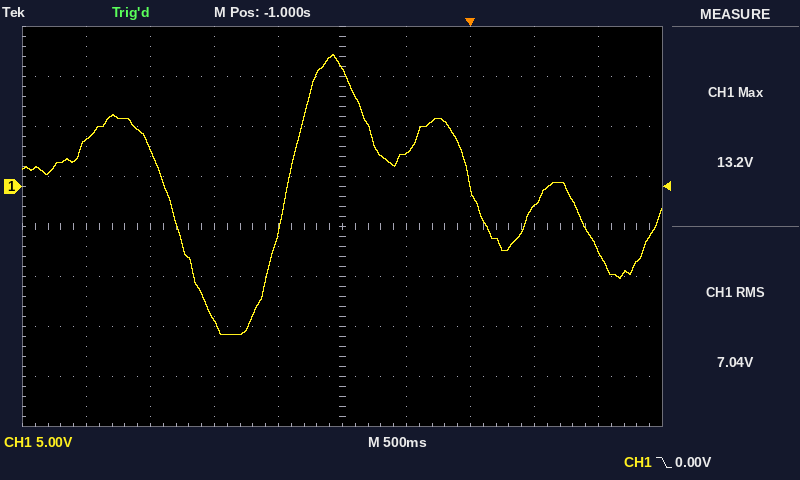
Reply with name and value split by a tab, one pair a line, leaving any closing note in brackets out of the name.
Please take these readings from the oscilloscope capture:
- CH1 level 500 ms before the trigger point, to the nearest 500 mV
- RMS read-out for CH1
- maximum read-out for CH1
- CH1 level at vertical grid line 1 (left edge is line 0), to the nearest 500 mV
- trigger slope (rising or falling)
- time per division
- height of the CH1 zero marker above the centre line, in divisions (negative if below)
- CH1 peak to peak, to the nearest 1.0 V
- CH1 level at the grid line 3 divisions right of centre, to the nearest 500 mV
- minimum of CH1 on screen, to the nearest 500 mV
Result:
CH1 level 500 ms before the trigger point, to the nearest 500 mV	3.5 V
RMS read-out for CH1	7.04 V
maximum read-out for CH1	13.2 V
CH1 level at vertical grid line 1 (left edge is line 0), to the nearest 500 mV	4.5 V
trigger slope	falling
time per division	500 ms
height of the CH1 zero marker above the centre line, in divisions	+0.8 div
CH1 peak to peak, to the nearest 1.0 V	28.0 V
CH1 level at the grid line 3 divisions right of centre, to the nearest 500 mV	-2.0 V
minimum of CH1 on screen, to the nearest 500 mV	-15.0 V
